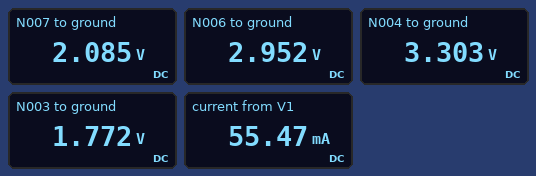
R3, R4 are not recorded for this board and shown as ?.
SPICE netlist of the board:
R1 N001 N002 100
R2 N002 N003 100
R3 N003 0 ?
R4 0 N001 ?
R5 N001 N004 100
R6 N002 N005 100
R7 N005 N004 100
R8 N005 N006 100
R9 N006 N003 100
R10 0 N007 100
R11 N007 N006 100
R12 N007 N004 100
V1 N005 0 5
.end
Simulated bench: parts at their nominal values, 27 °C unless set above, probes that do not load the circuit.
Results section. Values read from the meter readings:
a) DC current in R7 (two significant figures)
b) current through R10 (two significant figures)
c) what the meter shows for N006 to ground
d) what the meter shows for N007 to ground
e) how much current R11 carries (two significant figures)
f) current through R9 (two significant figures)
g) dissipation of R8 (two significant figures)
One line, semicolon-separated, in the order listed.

17 mA; 21 mA; 2.952 V; 2.085 V; 8.7 mA; 12 mA; 42 mW
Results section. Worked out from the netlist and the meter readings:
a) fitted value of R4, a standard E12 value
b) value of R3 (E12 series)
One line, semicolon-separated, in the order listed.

330 Ω; 68 Ω
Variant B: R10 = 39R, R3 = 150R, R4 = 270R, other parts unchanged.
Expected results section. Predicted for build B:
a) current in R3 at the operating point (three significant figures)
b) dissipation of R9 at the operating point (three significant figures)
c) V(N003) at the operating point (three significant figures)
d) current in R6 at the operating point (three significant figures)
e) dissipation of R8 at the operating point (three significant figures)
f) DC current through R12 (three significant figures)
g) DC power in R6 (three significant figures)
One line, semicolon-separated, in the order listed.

15.5 mA; 2.97 mW; 2.32 V; 16.7 mA; 45.4 mW; 17.0 mA; 27.9 mW
